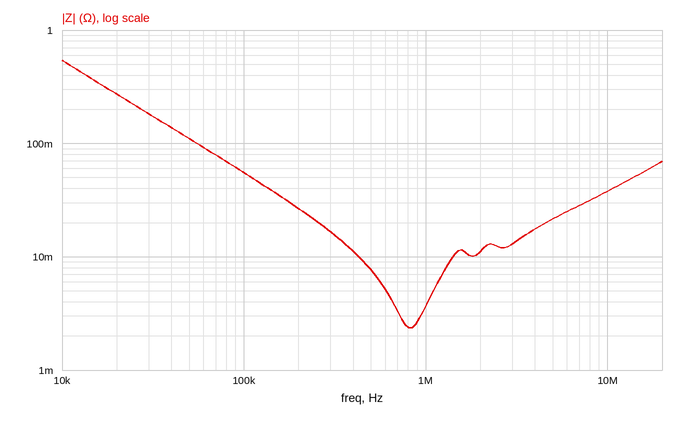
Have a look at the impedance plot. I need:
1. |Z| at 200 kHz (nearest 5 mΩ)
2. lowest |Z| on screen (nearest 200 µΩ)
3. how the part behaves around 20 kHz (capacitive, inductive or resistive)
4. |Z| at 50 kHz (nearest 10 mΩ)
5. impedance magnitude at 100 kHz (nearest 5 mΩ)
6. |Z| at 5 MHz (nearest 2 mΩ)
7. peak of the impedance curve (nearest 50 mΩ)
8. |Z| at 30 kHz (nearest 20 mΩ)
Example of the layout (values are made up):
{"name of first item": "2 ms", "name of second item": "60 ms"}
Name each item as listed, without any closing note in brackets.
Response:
{"|Z| at 200 kHz": "25 mΩ", "lowest |Z| on screen": "2.4 mΩ", "how the part behaves around 20 kHz": "capacitive", "|Z| at 50 kHz": "110 mΩ", "impedance magnitude at 100 kHz": "55 mΩ", "|Z| at 5 MHz": "22 mΩ", "peak of the impedance curve": "550 mΩ", "|Z| at 30 kHz": "180 mΩ"}
